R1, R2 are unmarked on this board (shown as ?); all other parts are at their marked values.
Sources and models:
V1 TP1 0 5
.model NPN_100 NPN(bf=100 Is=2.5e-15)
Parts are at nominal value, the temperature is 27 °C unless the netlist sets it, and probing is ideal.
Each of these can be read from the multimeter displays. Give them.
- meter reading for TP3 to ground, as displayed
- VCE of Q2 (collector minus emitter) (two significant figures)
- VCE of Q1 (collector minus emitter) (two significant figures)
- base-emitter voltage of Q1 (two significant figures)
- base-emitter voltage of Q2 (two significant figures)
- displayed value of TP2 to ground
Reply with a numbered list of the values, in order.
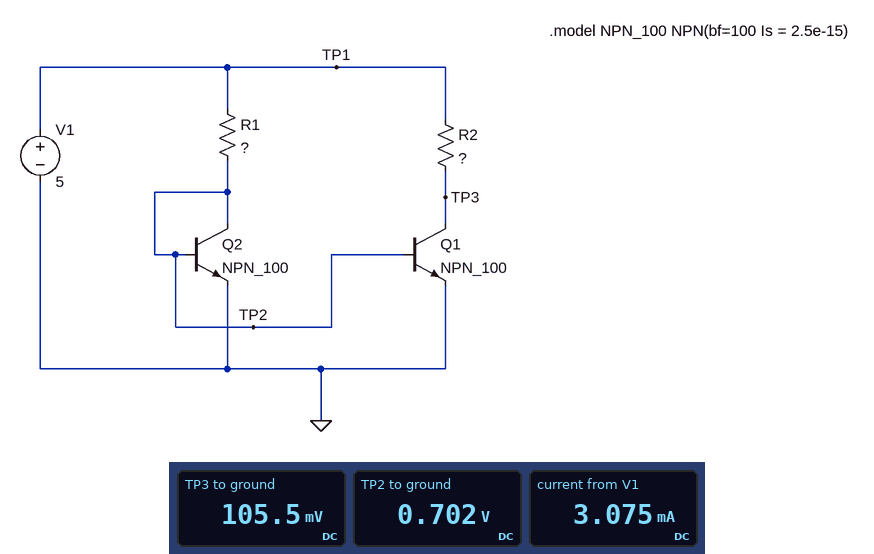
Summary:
1. 105.5 mV
2. 700 mV
3. 110 mV
4. 700 mV
5. 700 mV
6. 0.702 V
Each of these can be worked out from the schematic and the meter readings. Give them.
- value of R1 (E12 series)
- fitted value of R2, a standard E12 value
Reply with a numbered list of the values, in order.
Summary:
1. 2.7 kΩ
2. 3.3 kΩ
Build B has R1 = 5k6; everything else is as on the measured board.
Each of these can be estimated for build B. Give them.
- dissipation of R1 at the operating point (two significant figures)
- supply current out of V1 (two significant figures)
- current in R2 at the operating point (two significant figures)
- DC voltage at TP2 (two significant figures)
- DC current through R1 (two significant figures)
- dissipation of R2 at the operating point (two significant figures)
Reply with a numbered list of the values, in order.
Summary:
1. 3.3 mW
2. 1.5 mA
3. 760 µA
4. 680 mV
5. 770 µA
6. 1.9 mW
